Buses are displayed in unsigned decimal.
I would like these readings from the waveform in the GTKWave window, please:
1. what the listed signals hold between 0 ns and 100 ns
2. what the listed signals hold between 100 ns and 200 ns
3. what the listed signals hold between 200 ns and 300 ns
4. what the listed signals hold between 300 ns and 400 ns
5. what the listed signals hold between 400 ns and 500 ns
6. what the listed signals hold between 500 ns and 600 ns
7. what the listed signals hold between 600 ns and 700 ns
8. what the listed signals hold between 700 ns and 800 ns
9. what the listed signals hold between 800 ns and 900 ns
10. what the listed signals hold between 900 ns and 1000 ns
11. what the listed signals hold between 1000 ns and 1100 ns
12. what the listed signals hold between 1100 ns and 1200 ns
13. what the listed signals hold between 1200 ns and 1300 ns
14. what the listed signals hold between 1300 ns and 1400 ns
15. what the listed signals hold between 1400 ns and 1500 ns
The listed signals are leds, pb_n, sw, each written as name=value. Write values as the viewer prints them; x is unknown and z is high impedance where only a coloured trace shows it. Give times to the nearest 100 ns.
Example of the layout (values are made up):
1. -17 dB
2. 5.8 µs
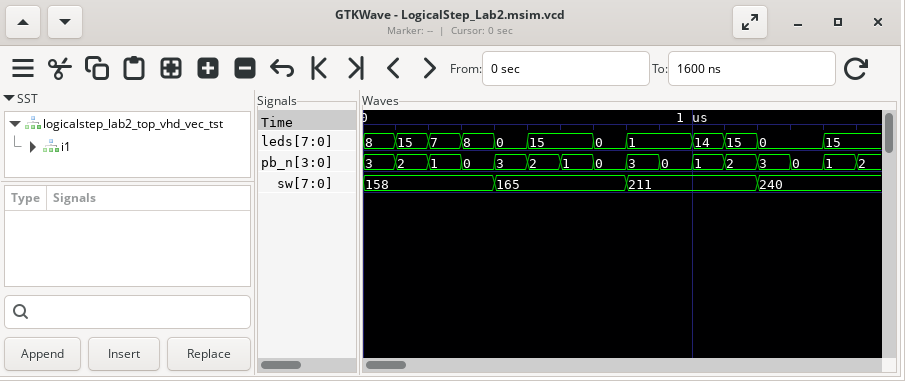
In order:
1. leds=8, pb_n=3, sw=158
2. leds=15, pb_n=2, sw=158
3. leds=7, pb_n=1, sw=158
4. leds=8, pb_n=0, sw=158
5. leds=0, pb_n=3, sw=165
6. leds=15, pb_n=2, sw=165
7. leds=15, pb_n=1, sw=165
8. leds=0, pb_n=0, sw=165
9. leds=1, pb_n=3, sw=211
10. leds=1, pb_n=0, sw=211
11. leds=14, pb_n=1, sw=211
12. leds=15, pb_n=2, sw=211
13. leds=0, pb_n=3, sw=240
14. leds=0, pb_n=0, sw=240
15. leds=15, pb_n=1, sw=240
